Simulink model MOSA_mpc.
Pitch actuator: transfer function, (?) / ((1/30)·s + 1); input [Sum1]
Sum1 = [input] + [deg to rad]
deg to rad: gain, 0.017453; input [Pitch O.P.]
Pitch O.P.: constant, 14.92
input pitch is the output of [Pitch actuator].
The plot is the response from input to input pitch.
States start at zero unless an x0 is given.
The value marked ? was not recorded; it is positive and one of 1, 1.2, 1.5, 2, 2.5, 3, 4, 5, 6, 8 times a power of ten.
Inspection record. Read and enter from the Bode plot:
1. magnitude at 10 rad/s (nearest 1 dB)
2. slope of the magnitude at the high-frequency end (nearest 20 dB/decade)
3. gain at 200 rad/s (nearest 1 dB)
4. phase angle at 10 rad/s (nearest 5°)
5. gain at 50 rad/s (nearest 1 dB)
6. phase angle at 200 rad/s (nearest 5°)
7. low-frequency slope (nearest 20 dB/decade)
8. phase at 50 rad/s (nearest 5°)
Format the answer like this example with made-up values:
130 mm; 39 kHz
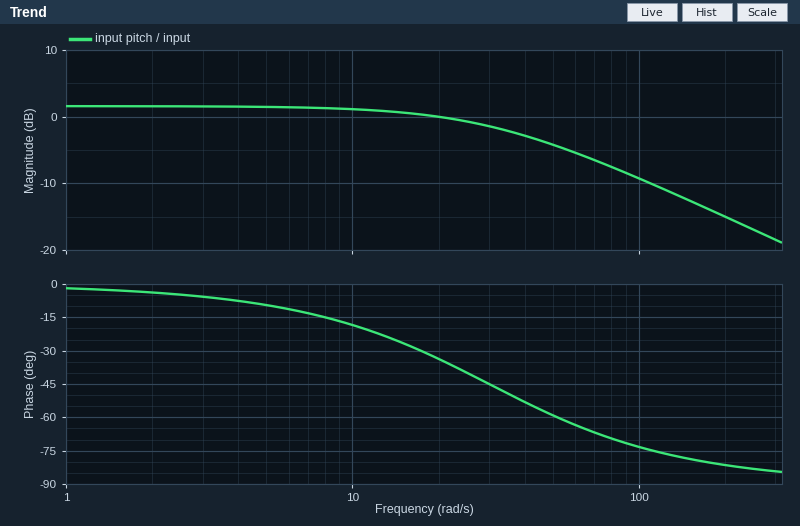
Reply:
1 dB; -20 dB/decade; -15 dB; -20°; -4 dB; -80°; 0 dB/decade; -60°
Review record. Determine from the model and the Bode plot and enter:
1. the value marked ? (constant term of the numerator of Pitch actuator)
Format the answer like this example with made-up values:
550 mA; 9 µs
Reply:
1.2
